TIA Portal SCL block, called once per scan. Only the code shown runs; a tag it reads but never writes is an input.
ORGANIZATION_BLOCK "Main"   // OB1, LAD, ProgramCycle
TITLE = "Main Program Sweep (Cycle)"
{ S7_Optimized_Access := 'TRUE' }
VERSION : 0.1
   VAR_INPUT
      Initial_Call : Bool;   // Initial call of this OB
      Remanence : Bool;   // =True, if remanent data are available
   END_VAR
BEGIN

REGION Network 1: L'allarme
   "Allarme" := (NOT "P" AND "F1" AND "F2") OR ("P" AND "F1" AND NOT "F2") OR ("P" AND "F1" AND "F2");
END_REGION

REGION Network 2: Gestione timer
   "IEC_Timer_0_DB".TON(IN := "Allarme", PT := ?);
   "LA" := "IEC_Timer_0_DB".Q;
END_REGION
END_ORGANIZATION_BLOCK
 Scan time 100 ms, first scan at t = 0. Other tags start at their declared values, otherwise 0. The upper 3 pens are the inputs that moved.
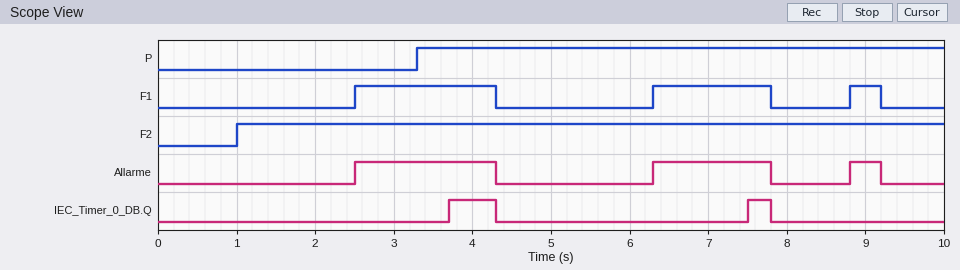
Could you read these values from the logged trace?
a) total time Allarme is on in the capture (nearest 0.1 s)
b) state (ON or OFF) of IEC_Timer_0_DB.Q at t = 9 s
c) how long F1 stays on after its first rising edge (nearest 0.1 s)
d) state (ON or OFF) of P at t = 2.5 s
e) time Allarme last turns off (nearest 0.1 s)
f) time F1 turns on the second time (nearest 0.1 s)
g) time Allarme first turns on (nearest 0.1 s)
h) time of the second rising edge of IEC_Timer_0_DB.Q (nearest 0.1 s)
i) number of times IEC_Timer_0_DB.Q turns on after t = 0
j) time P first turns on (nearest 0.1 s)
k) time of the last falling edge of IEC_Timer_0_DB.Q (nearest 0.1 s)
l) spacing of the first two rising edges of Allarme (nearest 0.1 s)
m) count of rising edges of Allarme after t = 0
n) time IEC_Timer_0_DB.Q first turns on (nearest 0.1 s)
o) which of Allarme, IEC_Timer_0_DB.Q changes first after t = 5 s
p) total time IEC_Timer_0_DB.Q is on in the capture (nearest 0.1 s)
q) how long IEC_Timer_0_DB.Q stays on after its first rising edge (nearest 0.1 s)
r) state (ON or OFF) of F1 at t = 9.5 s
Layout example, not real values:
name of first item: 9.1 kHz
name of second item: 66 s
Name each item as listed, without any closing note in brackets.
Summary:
total time Allarme is on in the capture: 3.7 s
state (ON or OFF) of IEC_Timer_0_DB.Q at t = 9 s: OFF
how long F1 stays on after its first rising edge: 1.8 s
state (ON or OFF) of P at t = 2.5 s: OFF
time Allarme last turns off: 9.2 s
time F1 turns on the second time: 6.3 s
time Allarme first turns on: 2.5 s
time of the second rising edge of IEC_Timer_0_DB.Q: 7.5 s
number of times IEC_Timer_0_DB.Q turns on after t = 0: 2
time P first turns on: 3.3 s
time of the last falling edge of IEC_Timer_0_DB.Q: 7.8 s
spacing of the first two rising edges of Allarme: 3.8 s
count of rising edges of Allarme after t = 0: 3
time IEC_Timer_0_DB.Q first turns on: 3.7 s
which of Allarme, IEC_Timer_0_DB.Q changes first after t = 5 s: Allarme
total time IEC_Timer_0_DB.Q is on in the capture: 0.9 s
how long IEC_Timer_0_DB.Q stays on after its first rising edge: 0.6 s
state (ON or OFF) of F1 at t = 9.5 s: OFF
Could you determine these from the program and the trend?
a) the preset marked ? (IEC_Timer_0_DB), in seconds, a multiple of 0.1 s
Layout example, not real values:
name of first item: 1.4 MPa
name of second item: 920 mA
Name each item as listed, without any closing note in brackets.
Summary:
the preset marked ? (IEC_Timer_0_DB), in seconds, a multiple of 0.1 s: 1.2 s
